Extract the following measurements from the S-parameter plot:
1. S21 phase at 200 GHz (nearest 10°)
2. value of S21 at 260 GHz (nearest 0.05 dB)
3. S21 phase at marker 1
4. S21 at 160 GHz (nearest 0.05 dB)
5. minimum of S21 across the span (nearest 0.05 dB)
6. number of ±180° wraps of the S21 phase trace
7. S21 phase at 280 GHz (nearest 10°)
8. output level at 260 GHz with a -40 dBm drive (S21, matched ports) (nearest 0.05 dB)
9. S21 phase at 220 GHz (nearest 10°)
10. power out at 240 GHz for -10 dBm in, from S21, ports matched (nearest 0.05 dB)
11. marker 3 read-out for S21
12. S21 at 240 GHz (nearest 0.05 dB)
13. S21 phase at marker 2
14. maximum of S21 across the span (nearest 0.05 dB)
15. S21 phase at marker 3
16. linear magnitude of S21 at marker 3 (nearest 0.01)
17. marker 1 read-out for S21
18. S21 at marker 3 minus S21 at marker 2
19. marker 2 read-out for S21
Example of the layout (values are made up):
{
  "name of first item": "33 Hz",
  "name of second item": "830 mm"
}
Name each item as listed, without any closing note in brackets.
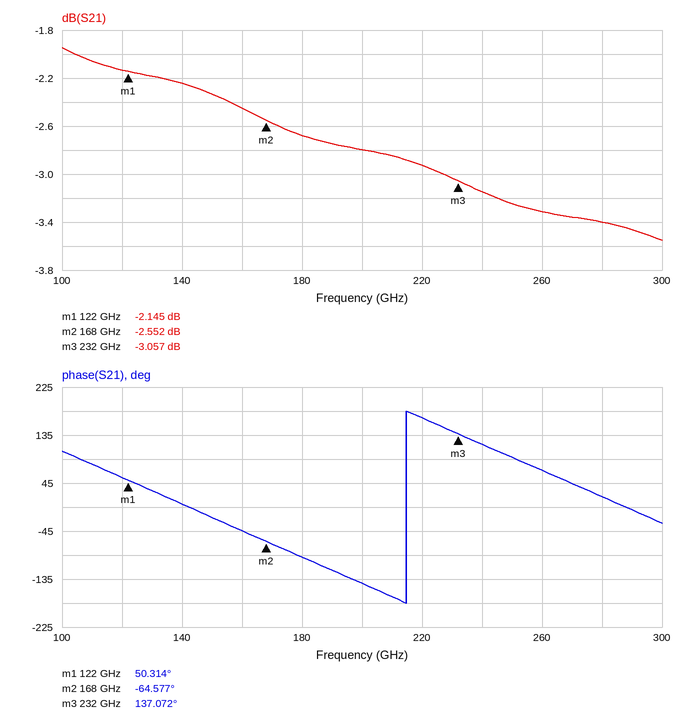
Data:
{
  "S21 phase at 200 GHz": "-140°",
  "value of S21 at 260 GHz": "-3.30 dB",
  "S21 phase at marker 1": "50.314°",
  "S21 at 160 GHz": "-2.45 dB",
  "minimum of S21 across the span": "-3.55 dB",
  "number of ±180° wraps of the S21 phase trace": "1",
  "S21 phase at 280 GHz": "20°",
  "output level at 260 GHz with a -40 dBm drive (S21, matched ports)": "-43.30 dBm",
  "S21 phase at 220 GHz": "170°",
  "power out at 240 GHz for -10 dBm in, from S21, ports matched": "-13.15 dBm",
  "marker 3 read-out for S21": "-3.057 dB",
  "S21 at 240 GHz": "-3.15 dB",
  "S21 phase at marker 2": "-64.577°",
  "maximum of S21 across the span": "-1.95 dB",
  "S21 phase at marker 3": "137.072°",
  "linear magnitude of S21 at marker 3": "0.70",
  "marker 1 read-out for S21": "-2.145 dB",
  "S21 at marker 3 minus S21 at marker 2": "-0.505 dB",
  "marker 2 read-out for S21": "-2.552 dB"
}
